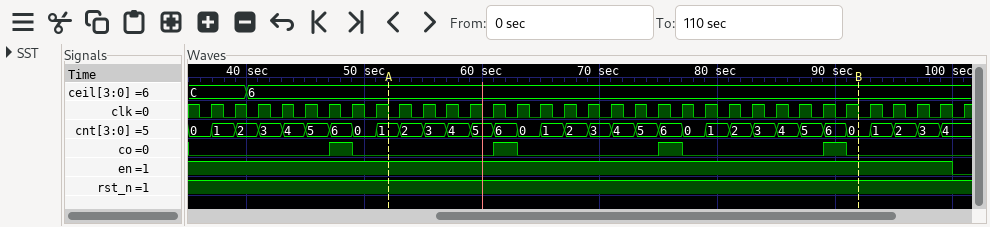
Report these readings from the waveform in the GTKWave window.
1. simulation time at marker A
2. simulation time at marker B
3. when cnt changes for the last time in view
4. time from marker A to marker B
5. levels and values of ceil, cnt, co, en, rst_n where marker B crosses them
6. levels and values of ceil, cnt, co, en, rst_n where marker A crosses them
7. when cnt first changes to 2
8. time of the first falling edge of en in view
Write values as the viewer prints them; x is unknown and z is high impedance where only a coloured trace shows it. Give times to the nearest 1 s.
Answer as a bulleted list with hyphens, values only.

- 52 s
- 92 s
- 99 s
- 40 s
- ceil=6, cnt=0, co=0, en=1, rst_n=1
- ceil=6, cnt=1, co=0, en=1, rst_n=1
- 39 s
- 100 s
